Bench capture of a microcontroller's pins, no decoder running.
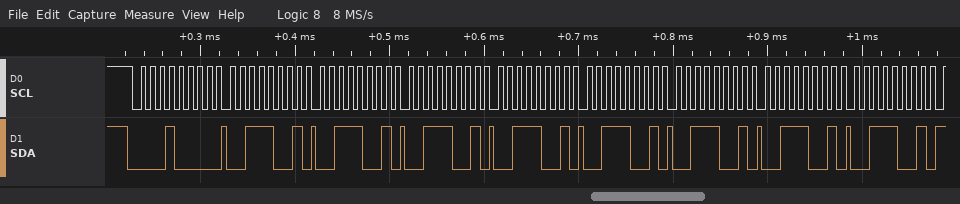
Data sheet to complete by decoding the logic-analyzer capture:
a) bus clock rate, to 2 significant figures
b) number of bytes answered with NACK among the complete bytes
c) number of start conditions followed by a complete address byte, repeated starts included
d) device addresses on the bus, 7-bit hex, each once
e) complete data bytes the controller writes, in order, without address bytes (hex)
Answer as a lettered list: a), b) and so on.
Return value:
a) 100 kHz
b) 0
c) 1
d) 0x08
e) 39 39 39 39 39 39 39 39
